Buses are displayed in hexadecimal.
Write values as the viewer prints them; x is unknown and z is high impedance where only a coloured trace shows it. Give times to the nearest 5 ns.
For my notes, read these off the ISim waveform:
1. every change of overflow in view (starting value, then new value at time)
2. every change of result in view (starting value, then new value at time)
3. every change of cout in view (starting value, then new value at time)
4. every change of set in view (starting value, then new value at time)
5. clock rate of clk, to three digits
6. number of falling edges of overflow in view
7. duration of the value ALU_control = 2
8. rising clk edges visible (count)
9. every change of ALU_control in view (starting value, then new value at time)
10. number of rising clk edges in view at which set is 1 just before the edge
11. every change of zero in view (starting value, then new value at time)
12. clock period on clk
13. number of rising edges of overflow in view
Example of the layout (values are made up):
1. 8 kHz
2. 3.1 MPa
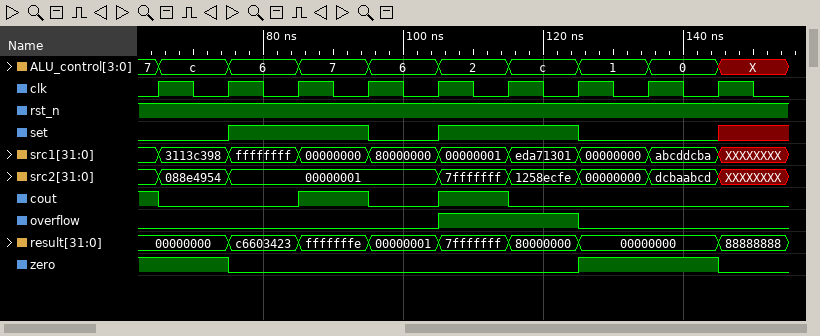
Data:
1. 0, 1 at 105 ns, 0 at 125 ns
2. 00000000, c6603423 at 75 ns, fffffffe at 85 ns, 00000001 at 95 ns, 7fffffff at 105 ns, 80000000 at 115 ns, 00000000 at 125 ns, 88888888 at 145 ns
3. 1, 0 at 65 ns, 1 at 85 ns, 0 at 95 ns, 1 at 105 ns, 0 at 115 ns
4. 0, 1 at 75 ns, 0 at 95 ns, 1 at 105 ns, 0 at 125 ns, x at 145 ns
5. 100 MHz
6. 1
7. 10 ns
8. 9
9. 7, c at 65 ns, 6 at 75 ns, 7 at 85 ns, 6 at 95 ns, 2 at 105 ns, c at 115 ns, 1 at 125 ns, 0 at 135 ns, X at 145 ns
10. 4
11. 1, 0 at 75 ns, 1 at 125 ns, 0 at 145 ns
12. 10 ns
13. 1
